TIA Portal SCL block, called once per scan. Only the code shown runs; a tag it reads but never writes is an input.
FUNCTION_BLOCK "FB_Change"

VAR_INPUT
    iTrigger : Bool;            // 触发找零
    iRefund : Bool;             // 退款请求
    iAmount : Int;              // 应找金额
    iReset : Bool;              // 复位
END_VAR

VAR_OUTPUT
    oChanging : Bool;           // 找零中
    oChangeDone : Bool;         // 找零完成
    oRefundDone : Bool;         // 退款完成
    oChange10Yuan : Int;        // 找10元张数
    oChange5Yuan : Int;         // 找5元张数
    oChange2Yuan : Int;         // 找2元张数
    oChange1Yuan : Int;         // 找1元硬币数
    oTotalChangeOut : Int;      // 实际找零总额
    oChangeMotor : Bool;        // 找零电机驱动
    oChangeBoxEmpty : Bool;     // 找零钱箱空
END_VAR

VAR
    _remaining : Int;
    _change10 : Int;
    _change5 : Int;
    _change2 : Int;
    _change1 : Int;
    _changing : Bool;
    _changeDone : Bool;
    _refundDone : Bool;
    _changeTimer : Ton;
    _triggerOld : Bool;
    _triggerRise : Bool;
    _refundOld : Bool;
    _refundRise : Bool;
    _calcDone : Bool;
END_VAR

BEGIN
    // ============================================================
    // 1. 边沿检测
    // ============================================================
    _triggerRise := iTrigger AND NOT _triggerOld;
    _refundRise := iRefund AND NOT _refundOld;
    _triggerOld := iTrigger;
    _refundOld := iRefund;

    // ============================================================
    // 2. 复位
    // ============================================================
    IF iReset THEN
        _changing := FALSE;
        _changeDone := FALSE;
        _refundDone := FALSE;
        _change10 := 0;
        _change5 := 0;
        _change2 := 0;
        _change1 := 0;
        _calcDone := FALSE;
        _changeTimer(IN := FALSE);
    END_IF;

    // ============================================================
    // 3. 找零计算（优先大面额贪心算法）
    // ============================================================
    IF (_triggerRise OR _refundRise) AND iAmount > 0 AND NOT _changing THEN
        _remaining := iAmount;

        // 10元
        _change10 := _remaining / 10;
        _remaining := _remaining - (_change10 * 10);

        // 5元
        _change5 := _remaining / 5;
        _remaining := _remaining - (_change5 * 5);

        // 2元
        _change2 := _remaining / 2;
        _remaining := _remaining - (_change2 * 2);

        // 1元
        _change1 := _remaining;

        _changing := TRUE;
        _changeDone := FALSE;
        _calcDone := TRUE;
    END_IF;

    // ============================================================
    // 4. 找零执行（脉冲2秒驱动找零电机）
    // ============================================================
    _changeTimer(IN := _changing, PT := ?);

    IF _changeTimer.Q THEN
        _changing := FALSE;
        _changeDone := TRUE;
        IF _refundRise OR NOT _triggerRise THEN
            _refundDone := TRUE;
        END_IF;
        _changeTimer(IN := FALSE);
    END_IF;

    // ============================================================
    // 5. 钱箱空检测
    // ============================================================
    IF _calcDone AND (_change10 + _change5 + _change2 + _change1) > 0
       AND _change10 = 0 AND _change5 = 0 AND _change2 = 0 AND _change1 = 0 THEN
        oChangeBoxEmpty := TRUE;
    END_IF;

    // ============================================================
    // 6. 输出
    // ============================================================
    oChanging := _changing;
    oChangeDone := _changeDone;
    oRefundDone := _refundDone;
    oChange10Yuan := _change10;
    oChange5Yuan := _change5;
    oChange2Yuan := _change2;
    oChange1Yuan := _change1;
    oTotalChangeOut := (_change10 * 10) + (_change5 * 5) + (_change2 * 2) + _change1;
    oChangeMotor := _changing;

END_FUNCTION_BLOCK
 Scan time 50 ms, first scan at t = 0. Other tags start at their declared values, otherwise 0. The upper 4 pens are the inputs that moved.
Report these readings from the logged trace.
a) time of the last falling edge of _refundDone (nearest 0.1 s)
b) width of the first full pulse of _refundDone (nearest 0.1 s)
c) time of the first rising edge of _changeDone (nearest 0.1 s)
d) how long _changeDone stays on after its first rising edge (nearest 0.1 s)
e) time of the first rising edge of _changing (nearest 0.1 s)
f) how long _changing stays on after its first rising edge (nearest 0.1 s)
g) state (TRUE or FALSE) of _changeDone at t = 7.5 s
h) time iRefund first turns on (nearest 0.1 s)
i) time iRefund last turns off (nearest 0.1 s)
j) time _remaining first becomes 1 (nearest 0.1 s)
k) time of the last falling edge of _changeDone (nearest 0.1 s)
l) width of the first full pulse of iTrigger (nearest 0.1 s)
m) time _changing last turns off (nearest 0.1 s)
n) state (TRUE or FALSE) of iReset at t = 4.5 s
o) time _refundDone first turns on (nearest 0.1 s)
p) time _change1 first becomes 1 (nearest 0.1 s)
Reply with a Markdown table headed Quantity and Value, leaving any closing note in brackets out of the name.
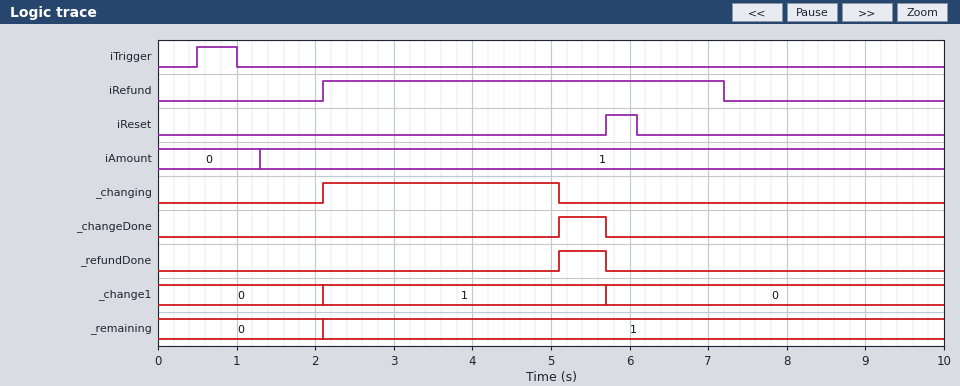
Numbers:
| Quantity | Value |
|---|---|
| time of the last falling edge of _refundDone | 5.7 s |
| width of the first full pulse of _refundDone | 0.6 s |
| time of the first rising edge of _changeDone | 5.1 s |
| how long _changeDone stays on after its first rising edge | 0.6 s |
| time of the first rising edge of _changing | 2.1 s |
| how long _changing stays on after its first rising edge | 3.0 s |
| state (TRUE or FALSE) of _changeDone at t = 7.5 s | FALSE |
| time iRefund first turns on | 2.1 s |
| time iRefund last turns off | 7.2 s |
| time _remaining first becomes 1 | 2.1 s |
| time of the last falling edge of _changeDone | 5.7 s |
| width of the first full pulse of iTrigger | 0.5 s |
| time _changing last turns off | 5.1 s |
| state (TRUE or FALSE) of iReset at t = 4.5 s | FALSE |
| time _refundDone first turns on | 5.1 s |
| time _change1 first becomes 1 | 2.1 s |
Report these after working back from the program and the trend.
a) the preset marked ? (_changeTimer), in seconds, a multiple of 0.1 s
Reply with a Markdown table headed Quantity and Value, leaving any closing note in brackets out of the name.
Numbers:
| Quantity | Value |
|---|---|
| the preset marked ? (_changeTimer), in seconds, a multiple of 0.1 s | 3.0 s |
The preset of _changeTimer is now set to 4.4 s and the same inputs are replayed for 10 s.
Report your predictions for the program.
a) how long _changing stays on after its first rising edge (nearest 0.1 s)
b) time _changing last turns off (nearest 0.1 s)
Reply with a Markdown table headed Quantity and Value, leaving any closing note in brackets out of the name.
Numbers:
| Quantity | Value |
|---|---|
| how long _changing stays on after its first rising edge | 3.6 s |
| time _changing last turns off | 5.7 s |
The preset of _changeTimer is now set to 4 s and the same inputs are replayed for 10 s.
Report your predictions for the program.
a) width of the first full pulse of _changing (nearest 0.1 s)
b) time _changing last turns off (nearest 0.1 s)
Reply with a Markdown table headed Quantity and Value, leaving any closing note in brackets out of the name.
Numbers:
| Quantity | Value |
|---|---|
| width of the first full pulse of _changing | 3.6 s |
| time _changing last turns off | 5.7 s |
